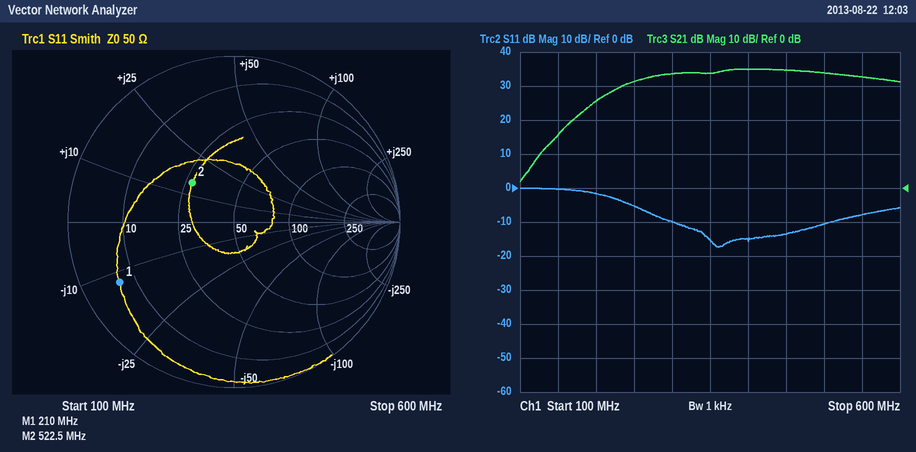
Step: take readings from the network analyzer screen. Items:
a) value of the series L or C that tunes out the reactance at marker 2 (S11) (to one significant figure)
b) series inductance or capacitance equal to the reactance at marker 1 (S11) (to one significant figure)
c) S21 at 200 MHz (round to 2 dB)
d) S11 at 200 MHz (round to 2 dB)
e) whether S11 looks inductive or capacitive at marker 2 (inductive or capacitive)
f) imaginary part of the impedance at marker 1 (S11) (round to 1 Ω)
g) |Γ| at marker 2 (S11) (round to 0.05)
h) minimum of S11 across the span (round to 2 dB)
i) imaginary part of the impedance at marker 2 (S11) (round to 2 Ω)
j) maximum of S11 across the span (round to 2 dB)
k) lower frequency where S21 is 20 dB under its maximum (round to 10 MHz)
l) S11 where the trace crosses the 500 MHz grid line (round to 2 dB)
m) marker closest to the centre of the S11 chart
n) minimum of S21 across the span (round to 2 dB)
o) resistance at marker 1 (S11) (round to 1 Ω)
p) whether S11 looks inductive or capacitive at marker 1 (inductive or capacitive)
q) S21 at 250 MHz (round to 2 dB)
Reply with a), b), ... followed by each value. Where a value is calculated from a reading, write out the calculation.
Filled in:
a) C = 1/(2π × 522.5 MHz × 14 Ω) ≈ 21.8 pF, so 20 pF to one significant figure
b) C = 1/(2π × 210 MHz × 12 Ω) ≈ 63.2 pF, so 60 pF to one significant figure
c) 26 dB
d) -2 dB
e) inductive
f) -12 Ω
g) 0.35
h) -18 dB
i) +14 Ω
j) 0 dB
k) 150 MHz
l) -10 dB
m) marker 2
n) 2 dB
o) 7 Ω
p) capacitive
q) 32 dB
